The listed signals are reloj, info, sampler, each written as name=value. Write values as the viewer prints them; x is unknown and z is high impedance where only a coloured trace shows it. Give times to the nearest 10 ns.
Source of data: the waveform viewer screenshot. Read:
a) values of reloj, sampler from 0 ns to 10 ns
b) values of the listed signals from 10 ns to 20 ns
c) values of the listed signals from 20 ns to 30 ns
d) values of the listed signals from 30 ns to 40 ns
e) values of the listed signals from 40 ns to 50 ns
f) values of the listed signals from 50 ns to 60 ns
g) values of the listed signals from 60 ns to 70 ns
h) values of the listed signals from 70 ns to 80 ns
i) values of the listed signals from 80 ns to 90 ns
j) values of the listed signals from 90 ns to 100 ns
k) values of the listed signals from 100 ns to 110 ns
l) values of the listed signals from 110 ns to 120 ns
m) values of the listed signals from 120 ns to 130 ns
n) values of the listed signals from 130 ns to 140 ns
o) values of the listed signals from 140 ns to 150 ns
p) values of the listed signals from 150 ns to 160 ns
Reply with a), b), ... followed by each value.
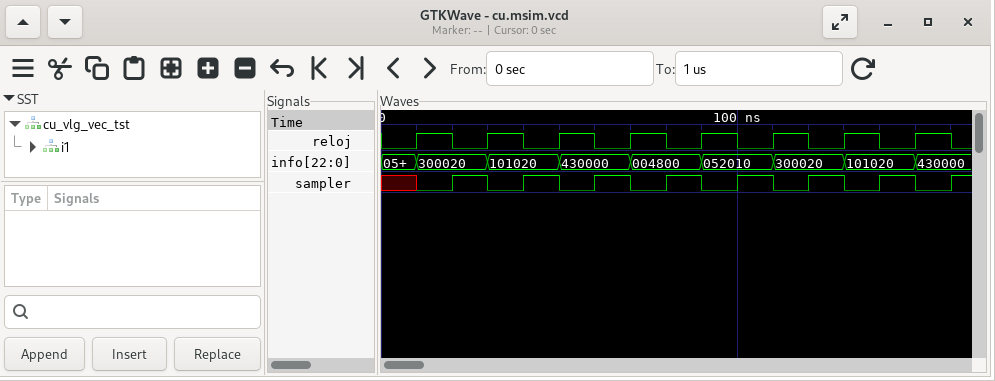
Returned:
a) reloj=0, sampler=x
b) reloj=1, info=300020, sampler=0
c) reloj=0, info=300020, sampler=1
d) reloj=1, info=101020, sampler=0
e) reloj=0, info=101020, sampler=1
f) reloj=1, info=430000, sampler=0
g) reloj=0, info=430000, sampler=1
h) reloj=1, info=004800, sampler=0
i) reloj=0, info=004800, sampler=1
j) reloj=1, info=052010, sampler=0
k) reloj=0, info=052010, sampler=1
l) reloj=1, info=300020, sampler=0
m) reloj=0, info=300020, sampler=1
n) reloj=1, info=101020, sampler=0
o) reloj=0, info=101020, sampler=1
p) reloj=1, info=430000, sampler=0
